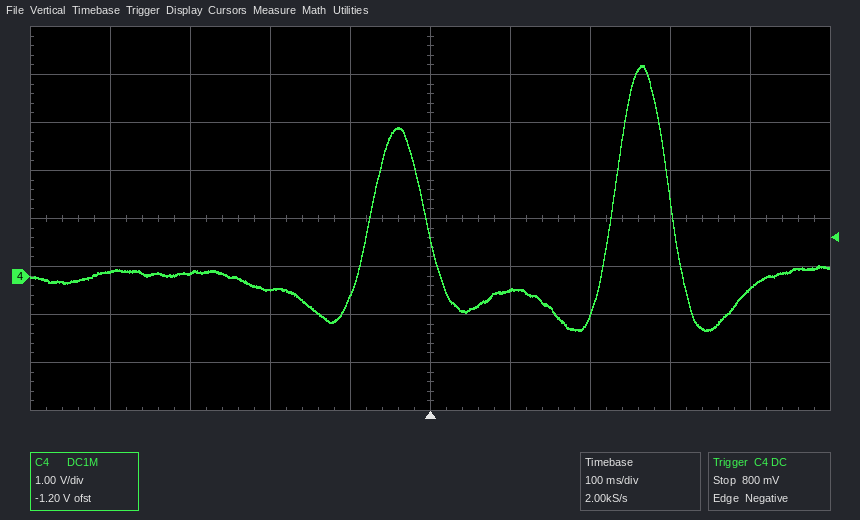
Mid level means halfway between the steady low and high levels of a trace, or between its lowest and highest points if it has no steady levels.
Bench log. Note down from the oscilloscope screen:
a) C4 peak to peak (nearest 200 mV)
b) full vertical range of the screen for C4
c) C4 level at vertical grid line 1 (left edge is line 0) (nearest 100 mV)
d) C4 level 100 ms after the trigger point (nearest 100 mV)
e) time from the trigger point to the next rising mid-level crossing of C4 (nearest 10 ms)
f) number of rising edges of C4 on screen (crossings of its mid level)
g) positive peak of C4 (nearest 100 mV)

5.6 V
8 V
100 mV
-300 mV
230 ms
2
4.4 V
